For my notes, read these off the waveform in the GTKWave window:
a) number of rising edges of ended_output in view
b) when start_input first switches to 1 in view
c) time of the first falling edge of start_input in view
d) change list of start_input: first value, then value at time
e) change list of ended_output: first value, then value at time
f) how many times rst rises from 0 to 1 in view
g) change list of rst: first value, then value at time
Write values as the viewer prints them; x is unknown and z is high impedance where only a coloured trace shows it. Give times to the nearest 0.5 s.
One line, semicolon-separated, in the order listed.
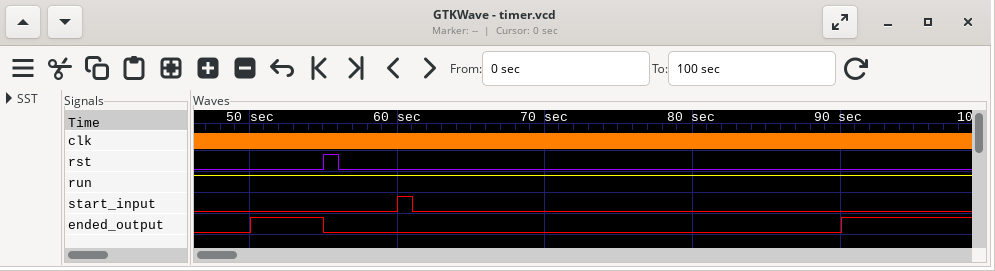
2; 60 s; 61 s; 0, 1 at 60 s, 0 at 61 s; 0, 1 at 50 s, 0 at 55 s, 1 at 90 s; 1; 0, 1 at 55 s, 0 at 56 s
